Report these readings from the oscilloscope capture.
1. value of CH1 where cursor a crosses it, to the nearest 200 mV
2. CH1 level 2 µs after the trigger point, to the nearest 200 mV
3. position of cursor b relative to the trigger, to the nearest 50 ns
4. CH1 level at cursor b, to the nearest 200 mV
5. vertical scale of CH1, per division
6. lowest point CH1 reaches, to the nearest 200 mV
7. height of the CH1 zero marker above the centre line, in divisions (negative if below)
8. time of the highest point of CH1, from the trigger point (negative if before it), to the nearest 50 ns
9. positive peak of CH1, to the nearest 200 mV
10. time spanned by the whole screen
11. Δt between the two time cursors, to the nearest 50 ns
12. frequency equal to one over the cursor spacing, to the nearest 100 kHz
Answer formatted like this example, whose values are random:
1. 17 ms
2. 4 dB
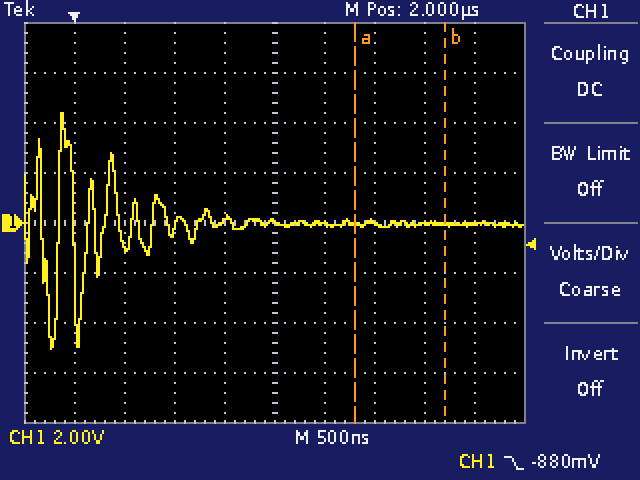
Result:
1. 0.0 V
2. 0.0 V
3. +3.70 µs
4. 0.0 V
5. 2 V
6. -5.0 V
7. 0.0 div
8. -100 ns
9. 4.4 V
10. 5 µs
11. 900 ns
12. 1.1 MHz
